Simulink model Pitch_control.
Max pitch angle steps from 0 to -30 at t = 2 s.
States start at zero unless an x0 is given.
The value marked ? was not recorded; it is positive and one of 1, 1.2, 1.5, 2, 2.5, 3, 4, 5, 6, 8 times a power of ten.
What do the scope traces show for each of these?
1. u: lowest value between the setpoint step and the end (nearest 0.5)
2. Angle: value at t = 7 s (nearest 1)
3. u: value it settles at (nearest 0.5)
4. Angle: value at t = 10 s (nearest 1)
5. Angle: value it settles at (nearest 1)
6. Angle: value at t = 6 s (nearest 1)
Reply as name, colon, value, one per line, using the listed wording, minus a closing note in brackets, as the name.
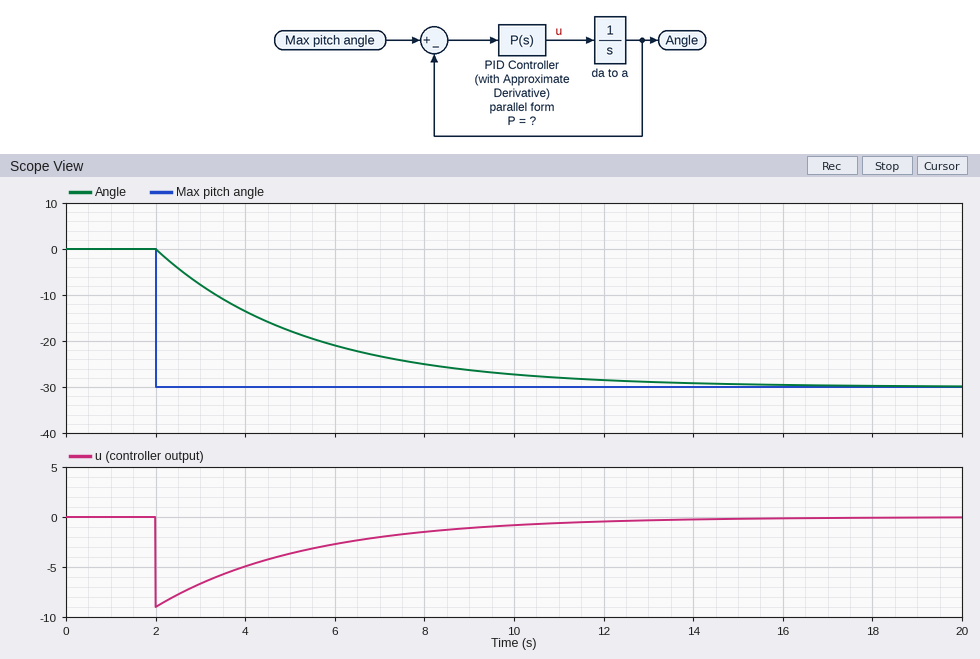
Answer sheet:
u: lowest value between the setpoint step and the end: -9.0
Angle: value at t = 7 s: -23
u: value it settles at: 0.0
Angle: value at t = 10 s: -27
Angle: value it settles at: -30
Angle: value at t = 6 s: -21
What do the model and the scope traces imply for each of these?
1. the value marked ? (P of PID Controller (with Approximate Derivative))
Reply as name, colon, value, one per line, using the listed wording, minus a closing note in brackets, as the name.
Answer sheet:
the value marked ? (P of PID Controller (with Approximate Derivative)): 0.3
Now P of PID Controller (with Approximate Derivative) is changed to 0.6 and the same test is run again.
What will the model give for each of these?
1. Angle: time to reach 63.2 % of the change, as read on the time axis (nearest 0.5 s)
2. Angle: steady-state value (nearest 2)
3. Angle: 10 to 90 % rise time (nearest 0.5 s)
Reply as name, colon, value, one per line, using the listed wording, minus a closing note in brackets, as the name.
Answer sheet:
Angle: time to reach 63.2 % of the change, as read on the time axis: 3.5 s
Angle: steady-state value: -30
Angle: 10 to 90 % rise time: 3.5 s
